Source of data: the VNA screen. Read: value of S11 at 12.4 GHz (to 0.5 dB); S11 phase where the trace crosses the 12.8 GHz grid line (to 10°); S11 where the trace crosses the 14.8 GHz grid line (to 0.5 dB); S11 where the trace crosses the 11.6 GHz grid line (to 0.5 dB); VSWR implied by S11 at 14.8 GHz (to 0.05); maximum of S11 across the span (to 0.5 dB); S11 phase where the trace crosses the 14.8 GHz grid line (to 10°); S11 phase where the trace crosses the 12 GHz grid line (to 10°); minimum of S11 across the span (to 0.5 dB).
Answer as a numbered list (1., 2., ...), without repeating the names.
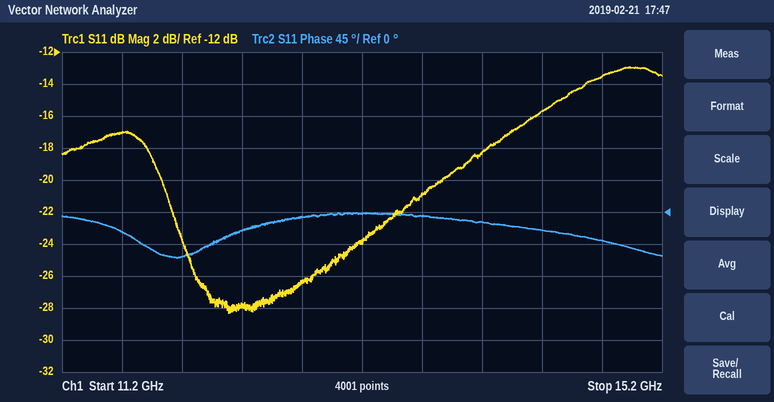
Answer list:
1. -28.0 dB
2. -10°
3. -13.5 dB
4. -17.0 dB
5. 1.55
6. -13.0 dB
7. -40°
8. -60°
9. -28.5 dB
